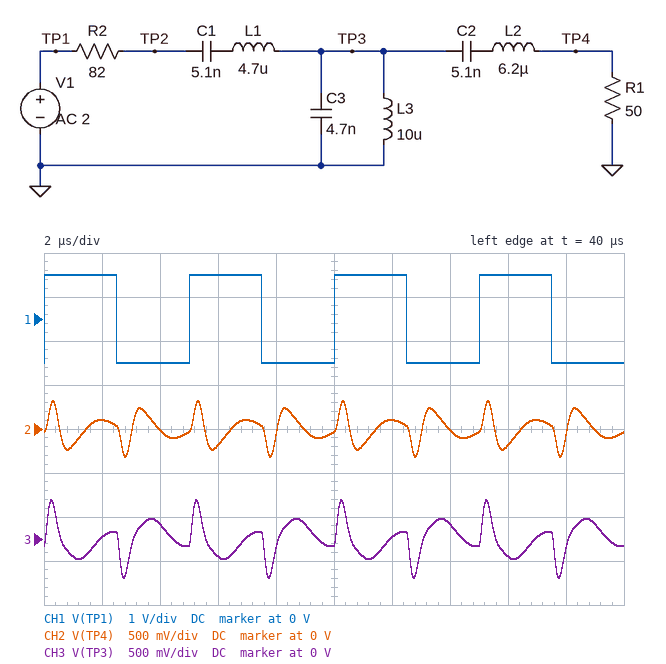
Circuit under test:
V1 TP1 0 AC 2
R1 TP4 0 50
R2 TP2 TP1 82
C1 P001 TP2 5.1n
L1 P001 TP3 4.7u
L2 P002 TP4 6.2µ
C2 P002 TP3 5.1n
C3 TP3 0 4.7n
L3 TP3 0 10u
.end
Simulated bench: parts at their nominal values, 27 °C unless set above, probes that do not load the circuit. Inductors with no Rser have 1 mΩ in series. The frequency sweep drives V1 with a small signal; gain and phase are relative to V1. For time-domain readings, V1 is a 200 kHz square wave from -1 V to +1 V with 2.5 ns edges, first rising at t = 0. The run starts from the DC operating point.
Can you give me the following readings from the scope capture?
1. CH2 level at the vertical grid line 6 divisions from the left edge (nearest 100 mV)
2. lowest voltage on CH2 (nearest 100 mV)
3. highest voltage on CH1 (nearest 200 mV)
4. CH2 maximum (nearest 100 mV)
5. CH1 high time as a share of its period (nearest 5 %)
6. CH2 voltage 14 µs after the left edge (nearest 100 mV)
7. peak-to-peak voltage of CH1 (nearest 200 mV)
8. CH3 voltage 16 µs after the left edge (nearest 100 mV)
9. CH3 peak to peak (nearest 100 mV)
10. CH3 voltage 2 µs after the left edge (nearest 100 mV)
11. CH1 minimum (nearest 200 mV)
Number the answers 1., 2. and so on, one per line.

1. 100 mV
2. -300 mV
3. 1.0 V
4. 300 mV
5. 50 %
6. 0 V
7. 2.0 V
8. -200 mV
9. 900 mV
10. 0 V
11. -1.0 V
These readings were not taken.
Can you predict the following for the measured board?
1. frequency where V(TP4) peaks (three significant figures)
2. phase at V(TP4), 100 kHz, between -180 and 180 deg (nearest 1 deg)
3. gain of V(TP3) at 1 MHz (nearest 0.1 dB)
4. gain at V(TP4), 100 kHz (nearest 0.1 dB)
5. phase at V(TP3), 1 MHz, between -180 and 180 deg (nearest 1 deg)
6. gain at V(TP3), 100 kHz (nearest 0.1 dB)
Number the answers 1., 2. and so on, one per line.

1. 517 kHz
2. -115 deg
3. -8.8 dB
4. -49.5 dB
5. -18 deg
6. -33.6 dB
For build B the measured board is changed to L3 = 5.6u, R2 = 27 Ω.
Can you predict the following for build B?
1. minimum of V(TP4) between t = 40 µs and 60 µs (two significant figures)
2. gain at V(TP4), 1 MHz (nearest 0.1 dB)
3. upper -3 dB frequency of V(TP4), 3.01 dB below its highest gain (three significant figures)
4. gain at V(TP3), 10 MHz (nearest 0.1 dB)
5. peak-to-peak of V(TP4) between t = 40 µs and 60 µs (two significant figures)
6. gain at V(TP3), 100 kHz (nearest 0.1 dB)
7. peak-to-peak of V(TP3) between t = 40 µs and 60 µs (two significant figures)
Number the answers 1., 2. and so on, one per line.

1. -560 mV
2. -3.8 dB
3. 1.99 MHz
4. -38.5 dB
5. 1.1 V
6. -38.6 dB
7. 1.7 V
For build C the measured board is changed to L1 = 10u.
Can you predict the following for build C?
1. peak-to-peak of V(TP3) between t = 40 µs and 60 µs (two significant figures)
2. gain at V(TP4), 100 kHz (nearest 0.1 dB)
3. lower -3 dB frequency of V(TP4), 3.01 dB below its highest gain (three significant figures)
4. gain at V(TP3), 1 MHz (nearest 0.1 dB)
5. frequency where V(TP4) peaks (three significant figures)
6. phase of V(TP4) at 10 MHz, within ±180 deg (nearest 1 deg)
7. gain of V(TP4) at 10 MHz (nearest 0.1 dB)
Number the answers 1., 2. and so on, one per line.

1. 830 mV
2. -49.4 dB
3. 380 kHz
4. -8.7 dB
5. 541 kHz
6. 105 deg
7. -63.1 dB
